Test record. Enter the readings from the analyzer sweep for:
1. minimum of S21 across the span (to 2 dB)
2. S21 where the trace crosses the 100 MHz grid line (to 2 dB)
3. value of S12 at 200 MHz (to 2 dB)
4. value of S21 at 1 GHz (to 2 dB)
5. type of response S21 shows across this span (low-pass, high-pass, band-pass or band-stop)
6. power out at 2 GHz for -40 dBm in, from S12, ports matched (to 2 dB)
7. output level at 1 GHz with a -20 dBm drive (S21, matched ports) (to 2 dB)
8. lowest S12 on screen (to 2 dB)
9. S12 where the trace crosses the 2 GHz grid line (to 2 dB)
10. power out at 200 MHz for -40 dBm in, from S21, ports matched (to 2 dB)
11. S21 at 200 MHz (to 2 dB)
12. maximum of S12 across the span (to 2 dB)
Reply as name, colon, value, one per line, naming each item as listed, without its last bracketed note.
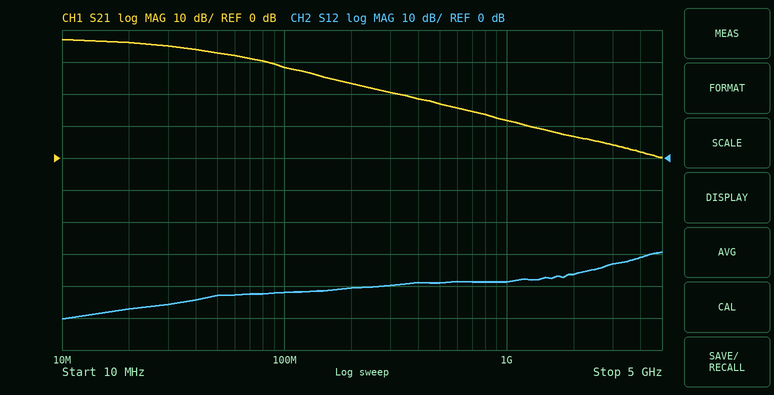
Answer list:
minimum of S21 across the span: 0 dB
S21 where the trace crosses the 100 MHz grid line: 28 dB
value of S12 at 200 MHz: -40 dB
value of S21 at 1 GHz: 12 dB
type of response S21 shows across this span: low-pass
power out at 2 GHz for -40 dBm in, from S12, ports matched: -76 dBm
output level at 1 GHz with a -20 dBm drive (S21, matched ports): -8 dBm
lowest S12 on screen: -50 dB
S12 where the trace crosses the 2 GHz grid line: -36 dB
power out at 200 MHz for -40 dBm in, from S21, ports matched: -16 dBm
S21 at 200 MHz: 24 dB
maximum of S12 across the span: -30 dB
